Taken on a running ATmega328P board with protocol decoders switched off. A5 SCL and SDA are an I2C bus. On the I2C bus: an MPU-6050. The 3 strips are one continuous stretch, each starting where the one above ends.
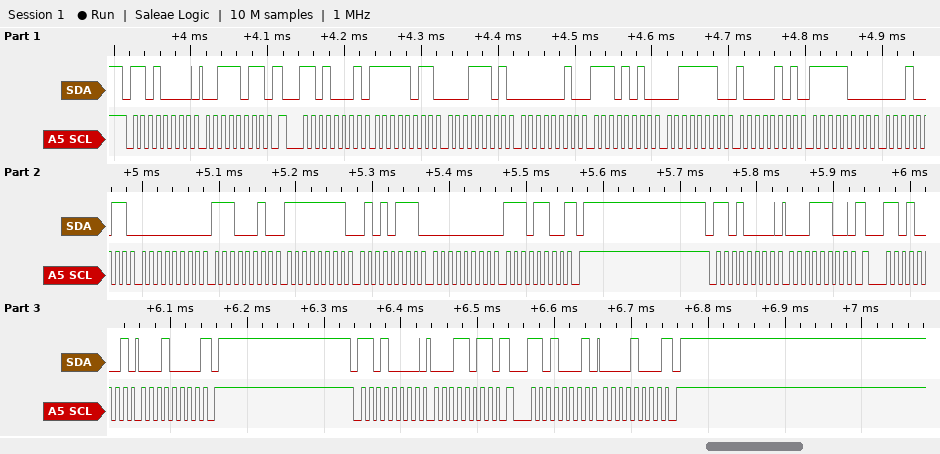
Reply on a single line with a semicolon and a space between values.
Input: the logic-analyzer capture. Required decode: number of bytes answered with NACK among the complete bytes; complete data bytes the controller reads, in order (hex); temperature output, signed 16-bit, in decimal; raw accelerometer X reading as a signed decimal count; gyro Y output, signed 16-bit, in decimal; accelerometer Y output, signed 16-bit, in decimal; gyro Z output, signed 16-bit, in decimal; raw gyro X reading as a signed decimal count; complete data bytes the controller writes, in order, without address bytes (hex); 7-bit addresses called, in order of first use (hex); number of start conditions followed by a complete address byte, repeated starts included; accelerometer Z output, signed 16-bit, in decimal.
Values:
3; FB 1D 02 EA 3E 85 F8 13 00 E2 FF 57 00 EC 10 08; -2029; -1251; -169; 746; 236; 226; 3B 1C 1B; 0x68; 6; 16005
